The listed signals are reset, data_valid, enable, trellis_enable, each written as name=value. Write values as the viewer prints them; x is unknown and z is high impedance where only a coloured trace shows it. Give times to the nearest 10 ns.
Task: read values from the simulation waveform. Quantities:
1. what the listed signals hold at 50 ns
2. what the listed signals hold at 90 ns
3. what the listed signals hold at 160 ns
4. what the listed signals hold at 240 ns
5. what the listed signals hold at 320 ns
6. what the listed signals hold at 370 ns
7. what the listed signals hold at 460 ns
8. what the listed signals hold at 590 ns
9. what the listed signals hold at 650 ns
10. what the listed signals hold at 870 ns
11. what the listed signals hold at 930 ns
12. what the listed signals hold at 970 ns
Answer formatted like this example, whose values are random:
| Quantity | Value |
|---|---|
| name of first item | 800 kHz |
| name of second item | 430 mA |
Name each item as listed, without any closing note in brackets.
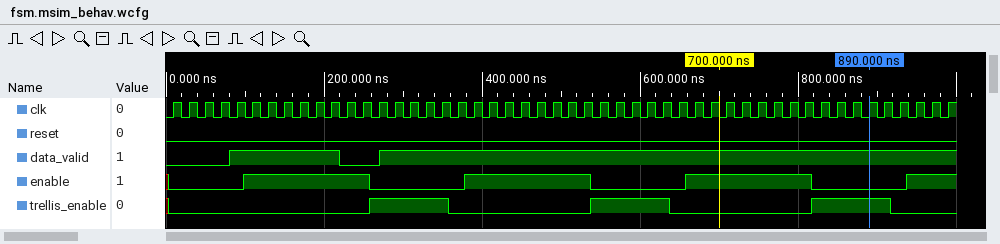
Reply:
| Quantity | Value |
|---|---|
| what the listed signals hold at 50 ns | reset=0, data_valid=0, enable=0, trellis_enable=0 |
| what the listed signals hold at 90 ns | reset=0, data_valid=1, enable=0, trellis_enable=0 |
| what the listed signals hold at 160 ns | reset=0, data_valid=1, enable=1, trellis_enable=0 |
| what the listed signals hold at 240 ns | reset=0, data_valid=0, enable=1, trellis_enable=0 |
| what the listed signals hold at 320 ns | reset=0, data_valid=1, enable=0, trellis_enable=1 |
| what the listed signals hold at 370 ns | reset=0, data_valid=1, enable=0, trellis_enable=0 |
| what the listed signals hold at 460 ns | reset=0, data_valid=1, enable=1, trellis_enable=0 |
| what the listed signals hold at 590 ns | reset=0, data_valid=1, enable=0, trellis_enable=1 |
| what the listed signals hold at 650 ns | reset=0, data_valid=1, enable=0, trellis_enable=0 |
| what the listed signals hold at 870 ns | reset=0, data_valid=1, enable=0, trellis_enable=1 |
| what the listed signals hold at 930 ns | reset=0, data_valid=1, enable=0, trellis_enable=0 |
| what the listed signals hold at 970 ns | reset=0, data_valid=1, enable=1, trellis_enable=0 |
